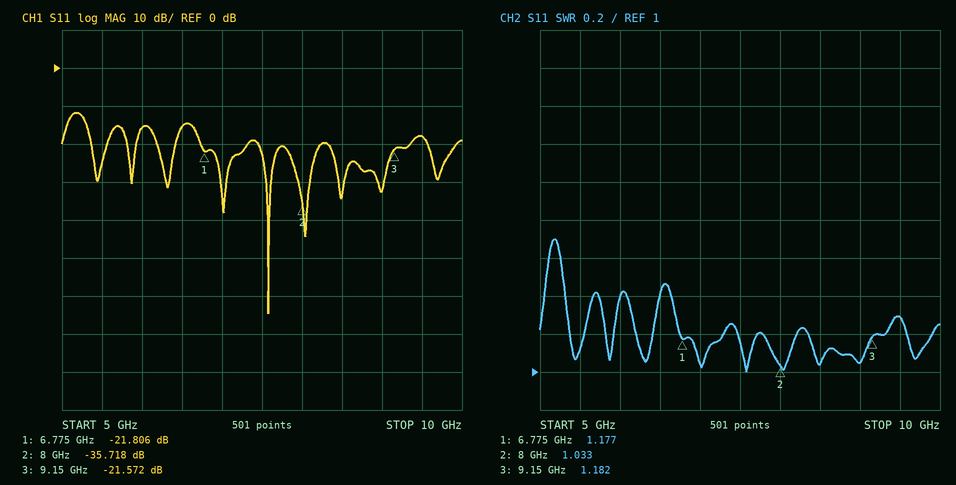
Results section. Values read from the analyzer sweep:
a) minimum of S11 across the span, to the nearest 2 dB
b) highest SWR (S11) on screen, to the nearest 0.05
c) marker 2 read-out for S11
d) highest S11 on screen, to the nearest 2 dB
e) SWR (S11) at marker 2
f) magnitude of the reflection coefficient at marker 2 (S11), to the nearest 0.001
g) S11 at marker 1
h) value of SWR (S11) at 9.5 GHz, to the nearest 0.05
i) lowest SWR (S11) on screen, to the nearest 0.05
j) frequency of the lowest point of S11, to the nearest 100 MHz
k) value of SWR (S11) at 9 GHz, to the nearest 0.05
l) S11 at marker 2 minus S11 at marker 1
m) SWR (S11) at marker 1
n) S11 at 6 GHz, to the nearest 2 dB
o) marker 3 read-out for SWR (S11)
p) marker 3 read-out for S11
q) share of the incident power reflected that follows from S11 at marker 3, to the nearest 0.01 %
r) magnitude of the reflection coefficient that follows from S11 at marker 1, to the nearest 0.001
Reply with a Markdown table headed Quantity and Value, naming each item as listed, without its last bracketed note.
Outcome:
| Quantity | Value |
|---|---|
| minimum of S11 across the span, to the nearest 2 dB | -64 dB |
| highest SWR (S11) on screen, to the nearest 0.05 | 1.70 |
| marker 2 read-out for S11 | -35.718 dB |
| highest S11 on screen, to the nearest 2 dB | -12 dB |
| SWR (S11) at marker 2 | 1.033 |
| magnitude of the reflection coefficient at marker 2 (S11), to the nearest 0.001 | 0.016 |
| S11 at marker 1 | -21.806 dB |
| value of SWR (S11) at 9.5 GHz, to the nearest 0.05 | 1.30 |
| lowest SWR (S11) on screen, to the nearest 0.05 | 1.00 |
| frequency of the lowest point of S11, to the nearest 100 MHz | 7.6 GHz |
| value of SWR (S11) at 9 GHz, to the nearest 0.05 | 1.05 |
| S11 at marker 2 minus S11 at marker 1 | -13.912 dB |
| SWR (S11) at marker 1 | 1.177 |
| S11 at 6 GHz, to the nearest 2 dB | -16 dB |
| marker 3 read-out for SWR | 1.182 |
| marker 3 read-out for S11 | -21.572 dB |
| share of the incident power reflected that follows from S11 at marker 3, to the nearest 0.01 % | 0.70 % |
| magnitude of the reflection coefficient that follows from S11 at marker 1, to the nearest 0.001 | 0.081 |
